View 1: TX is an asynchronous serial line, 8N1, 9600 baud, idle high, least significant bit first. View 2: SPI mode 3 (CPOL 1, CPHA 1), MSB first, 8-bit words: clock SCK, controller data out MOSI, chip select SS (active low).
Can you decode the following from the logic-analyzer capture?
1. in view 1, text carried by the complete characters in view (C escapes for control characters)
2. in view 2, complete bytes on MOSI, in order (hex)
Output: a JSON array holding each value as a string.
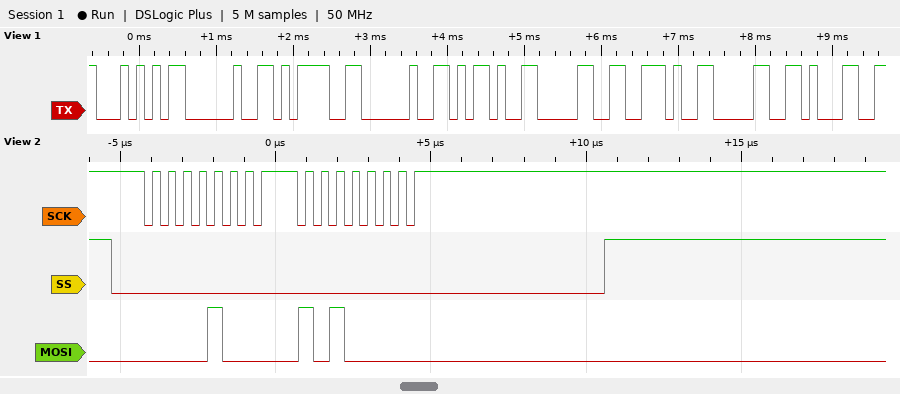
["\"T = -0.01\"", "08 A0"]
